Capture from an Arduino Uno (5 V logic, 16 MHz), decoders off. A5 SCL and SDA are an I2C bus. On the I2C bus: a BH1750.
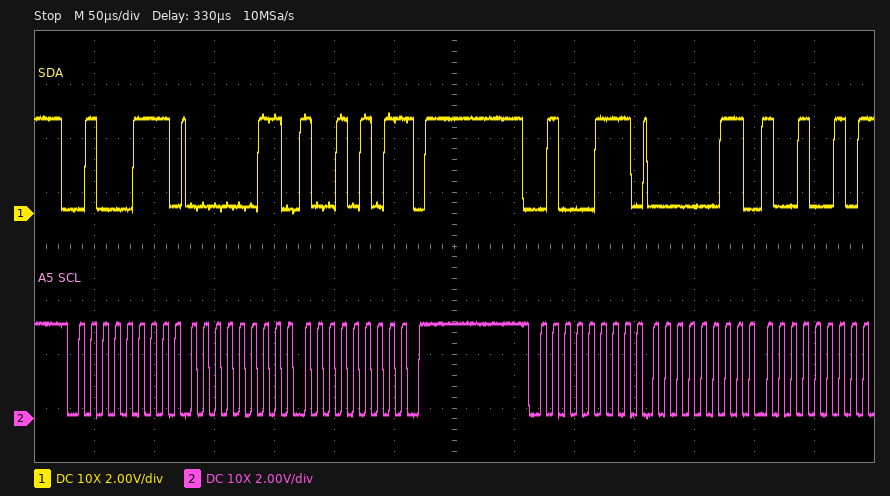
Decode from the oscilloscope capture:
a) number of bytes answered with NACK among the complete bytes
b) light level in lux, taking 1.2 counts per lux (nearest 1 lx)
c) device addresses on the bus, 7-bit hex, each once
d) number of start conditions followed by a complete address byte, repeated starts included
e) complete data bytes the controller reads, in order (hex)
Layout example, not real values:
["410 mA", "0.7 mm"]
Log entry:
["2", "764 lx", "0x23", "2", "03 95 03 92"]
